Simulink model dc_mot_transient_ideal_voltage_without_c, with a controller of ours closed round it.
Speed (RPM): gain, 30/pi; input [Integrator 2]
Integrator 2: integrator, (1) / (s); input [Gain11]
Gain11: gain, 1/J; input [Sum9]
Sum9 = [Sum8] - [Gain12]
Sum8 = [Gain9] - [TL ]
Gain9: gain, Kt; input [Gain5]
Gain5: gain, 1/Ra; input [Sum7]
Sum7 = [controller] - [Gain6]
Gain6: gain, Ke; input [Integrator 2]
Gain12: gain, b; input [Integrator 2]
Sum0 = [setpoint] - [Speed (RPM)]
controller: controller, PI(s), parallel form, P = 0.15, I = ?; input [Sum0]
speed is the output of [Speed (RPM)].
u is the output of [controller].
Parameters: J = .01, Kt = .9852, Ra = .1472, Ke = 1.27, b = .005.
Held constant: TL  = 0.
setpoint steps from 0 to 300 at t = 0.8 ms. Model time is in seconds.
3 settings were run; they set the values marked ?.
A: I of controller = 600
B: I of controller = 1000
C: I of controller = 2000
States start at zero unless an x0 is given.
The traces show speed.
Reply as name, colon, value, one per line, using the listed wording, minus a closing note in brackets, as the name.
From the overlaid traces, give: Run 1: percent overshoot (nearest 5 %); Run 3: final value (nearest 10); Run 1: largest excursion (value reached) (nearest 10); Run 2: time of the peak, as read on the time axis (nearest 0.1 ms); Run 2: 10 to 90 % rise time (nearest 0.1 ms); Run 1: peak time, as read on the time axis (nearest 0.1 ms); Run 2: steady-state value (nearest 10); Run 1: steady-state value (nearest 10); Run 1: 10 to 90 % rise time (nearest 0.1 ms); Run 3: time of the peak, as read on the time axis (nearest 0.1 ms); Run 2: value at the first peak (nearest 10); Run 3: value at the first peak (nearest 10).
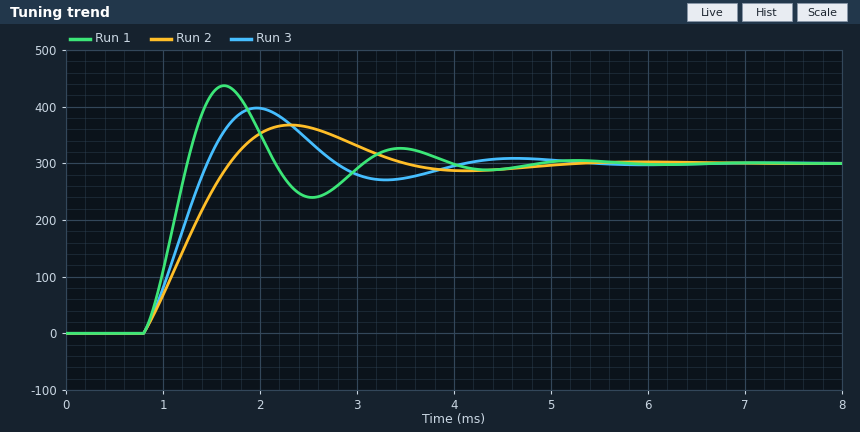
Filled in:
Run 1: percent overshoot: 45 %
Run 3: final value: 300
Run 1: largest excursion (value reached): 440
Run 2: time of the peak, as read on the time axis: 2.3 ms
Run 2: 10 to 90 % rise time: 0.7 ms
Run 1: peak time, as read on the time axis: 1.6 ms
Run 2: steady-state value: 300
Run 1: steady-state value: 300
Run 1: 10 to 90 % rise time: 0.3 ms
Run 3: time of the peak, as read on the time axis: 2.0 ms
Run 2: value at the first peak: 370
Run 3: value at the first peak: 400
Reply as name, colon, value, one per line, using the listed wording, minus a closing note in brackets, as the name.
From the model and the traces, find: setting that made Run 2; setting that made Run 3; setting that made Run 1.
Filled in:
setting that made Run 2: A
setting that made Run 3: B
setting that made Run 1: C
